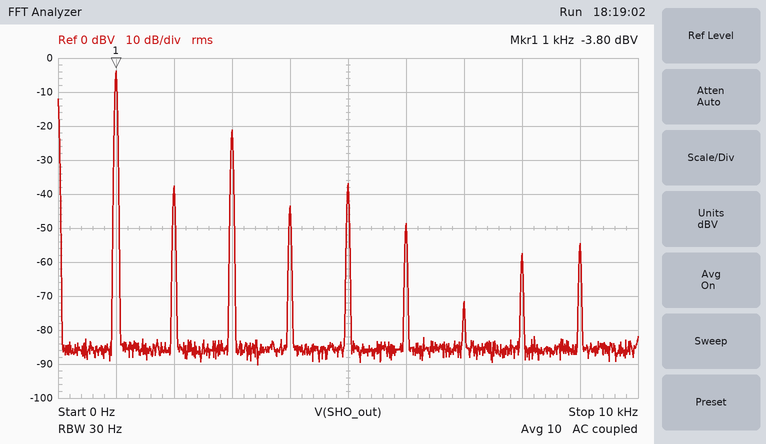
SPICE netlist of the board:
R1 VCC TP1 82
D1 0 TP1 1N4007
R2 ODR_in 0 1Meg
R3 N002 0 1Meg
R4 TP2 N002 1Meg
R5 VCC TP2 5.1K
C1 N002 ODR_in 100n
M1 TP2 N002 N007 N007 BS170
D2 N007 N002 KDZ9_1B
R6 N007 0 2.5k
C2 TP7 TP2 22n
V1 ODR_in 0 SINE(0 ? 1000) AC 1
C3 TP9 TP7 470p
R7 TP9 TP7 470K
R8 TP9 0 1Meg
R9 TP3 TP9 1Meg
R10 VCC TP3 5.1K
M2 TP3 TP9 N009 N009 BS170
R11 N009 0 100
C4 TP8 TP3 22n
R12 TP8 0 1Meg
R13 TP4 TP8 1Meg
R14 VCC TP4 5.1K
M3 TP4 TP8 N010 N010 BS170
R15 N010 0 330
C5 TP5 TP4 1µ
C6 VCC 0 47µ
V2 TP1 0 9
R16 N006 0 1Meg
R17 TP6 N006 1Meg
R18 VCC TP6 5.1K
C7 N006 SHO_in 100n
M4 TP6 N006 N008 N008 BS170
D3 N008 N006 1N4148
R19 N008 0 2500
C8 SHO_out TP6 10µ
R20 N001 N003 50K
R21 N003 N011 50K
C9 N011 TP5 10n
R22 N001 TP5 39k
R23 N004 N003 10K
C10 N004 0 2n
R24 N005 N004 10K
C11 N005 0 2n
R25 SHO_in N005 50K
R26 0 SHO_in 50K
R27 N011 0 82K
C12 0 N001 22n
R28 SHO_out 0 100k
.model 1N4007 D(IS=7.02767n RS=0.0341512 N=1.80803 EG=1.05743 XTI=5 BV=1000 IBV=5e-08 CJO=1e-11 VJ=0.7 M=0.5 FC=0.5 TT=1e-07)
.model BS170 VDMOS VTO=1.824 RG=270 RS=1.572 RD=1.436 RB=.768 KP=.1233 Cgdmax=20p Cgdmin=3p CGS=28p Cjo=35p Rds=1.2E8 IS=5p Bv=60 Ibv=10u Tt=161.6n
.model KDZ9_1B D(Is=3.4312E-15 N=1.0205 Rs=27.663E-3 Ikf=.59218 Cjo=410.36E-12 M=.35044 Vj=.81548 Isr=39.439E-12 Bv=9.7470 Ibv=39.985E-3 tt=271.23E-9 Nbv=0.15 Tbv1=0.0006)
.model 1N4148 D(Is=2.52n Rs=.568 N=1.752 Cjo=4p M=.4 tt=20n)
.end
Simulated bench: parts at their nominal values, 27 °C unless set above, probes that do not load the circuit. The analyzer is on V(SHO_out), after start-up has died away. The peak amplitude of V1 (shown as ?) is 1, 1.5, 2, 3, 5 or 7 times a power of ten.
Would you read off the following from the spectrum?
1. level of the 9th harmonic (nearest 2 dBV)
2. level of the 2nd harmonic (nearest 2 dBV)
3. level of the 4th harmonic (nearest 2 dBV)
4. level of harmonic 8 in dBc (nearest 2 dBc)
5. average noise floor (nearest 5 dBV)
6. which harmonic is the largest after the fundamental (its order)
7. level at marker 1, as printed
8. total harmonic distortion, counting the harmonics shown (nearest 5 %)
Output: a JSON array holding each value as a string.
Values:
["-54 dBV", "-38 dBV", "-44 dBV", "-54 dBc", "-85 dBV", "3", "-3.80 dBV", "15 %"]
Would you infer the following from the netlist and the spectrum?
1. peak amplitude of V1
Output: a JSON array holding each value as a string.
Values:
["150 mV"]
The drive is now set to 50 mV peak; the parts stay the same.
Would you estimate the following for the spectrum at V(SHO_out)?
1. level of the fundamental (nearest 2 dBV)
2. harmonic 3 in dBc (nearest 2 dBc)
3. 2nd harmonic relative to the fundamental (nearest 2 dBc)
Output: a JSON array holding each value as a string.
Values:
["-8 dBV", "-46 dBc", "-30 dBc"]
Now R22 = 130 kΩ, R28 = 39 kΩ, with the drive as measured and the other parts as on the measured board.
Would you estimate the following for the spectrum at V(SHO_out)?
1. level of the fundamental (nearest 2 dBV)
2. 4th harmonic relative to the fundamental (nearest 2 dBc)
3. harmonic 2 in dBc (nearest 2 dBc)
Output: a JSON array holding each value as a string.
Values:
["-4 dBV", "-54 dBc", "-38 dBc"]
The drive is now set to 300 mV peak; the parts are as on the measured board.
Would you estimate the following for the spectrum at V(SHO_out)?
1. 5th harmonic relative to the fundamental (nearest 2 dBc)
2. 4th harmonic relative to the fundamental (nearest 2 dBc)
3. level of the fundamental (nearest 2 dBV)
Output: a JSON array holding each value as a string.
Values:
["-24 dBc", "-42 dBc", "-4 dBV"]
